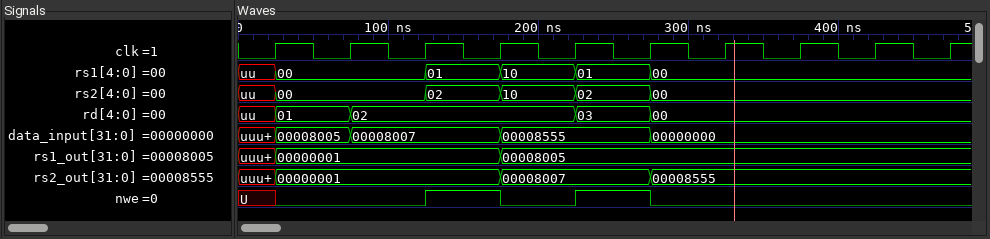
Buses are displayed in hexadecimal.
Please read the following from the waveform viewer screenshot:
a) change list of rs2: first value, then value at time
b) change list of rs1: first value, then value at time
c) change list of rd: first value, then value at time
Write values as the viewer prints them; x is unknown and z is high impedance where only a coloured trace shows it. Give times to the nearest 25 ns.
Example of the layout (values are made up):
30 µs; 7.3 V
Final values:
uu, 00 at 25 ns, 02 at 125 ns, 10 at 175 ns, 02 at 225 ns, 00 at 275 ns; uu, 00 at 25 ns, 01 at 125 ns, 10 at 175 ns, 01 at 225 ns, 00 at 275 ns; uu, 01 at 25 ns, 02 at 75 ns, 03 at 225 ns, 00 at 275 ns
